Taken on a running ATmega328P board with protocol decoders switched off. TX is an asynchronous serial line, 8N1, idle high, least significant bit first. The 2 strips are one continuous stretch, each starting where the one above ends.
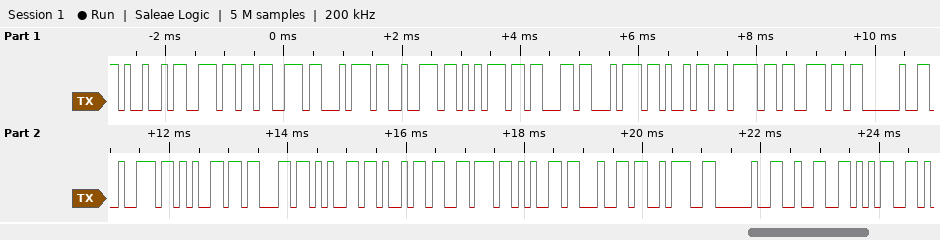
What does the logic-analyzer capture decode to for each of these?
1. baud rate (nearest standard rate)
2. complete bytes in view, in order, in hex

9600 baud
0x49 0x6E 0x73 0x74 0x72 0x75 0x63 0x74 0x69 0x6F 0x6E 0x20 0x72 0x65 0x63 0x65 0x69 0x76 0x65 0x64 0x3A 0x20 0x32 0x35
